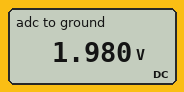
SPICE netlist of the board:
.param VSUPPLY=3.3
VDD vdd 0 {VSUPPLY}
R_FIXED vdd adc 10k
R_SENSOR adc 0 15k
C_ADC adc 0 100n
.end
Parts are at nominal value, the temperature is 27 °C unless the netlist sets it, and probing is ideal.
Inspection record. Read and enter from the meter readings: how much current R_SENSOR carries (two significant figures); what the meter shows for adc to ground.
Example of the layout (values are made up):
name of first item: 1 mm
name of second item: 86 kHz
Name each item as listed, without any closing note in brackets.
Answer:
how much current R_SENSOR carries: 130 µA
what the meter shows for adc to ground: 1.980 V
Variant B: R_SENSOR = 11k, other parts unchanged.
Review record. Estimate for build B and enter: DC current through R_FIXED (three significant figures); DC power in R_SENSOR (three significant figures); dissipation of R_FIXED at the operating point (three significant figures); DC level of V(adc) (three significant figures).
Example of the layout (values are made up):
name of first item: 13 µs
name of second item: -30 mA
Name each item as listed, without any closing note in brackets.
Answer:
DC current through R_FIXED: 157 µA
DC power in R_SENSOR: 272 µW
dissipation of R_FIXED at the operating point: 247 µW
DC level of V(adc): 1.73 V
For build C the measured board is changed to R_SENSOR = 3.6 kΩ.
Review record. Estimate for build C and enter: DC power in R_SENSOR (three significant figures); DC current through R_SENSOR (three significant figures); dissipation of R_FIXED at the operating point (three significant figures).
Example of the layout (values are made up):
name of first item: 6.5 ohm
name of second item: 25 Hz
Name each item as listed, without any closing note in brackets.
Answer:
DC power in R_SENSOR: 212 µW
DC current through R_SENSOR: 243 µA
dissipation of R_FIXED at the operating point: 589 µW
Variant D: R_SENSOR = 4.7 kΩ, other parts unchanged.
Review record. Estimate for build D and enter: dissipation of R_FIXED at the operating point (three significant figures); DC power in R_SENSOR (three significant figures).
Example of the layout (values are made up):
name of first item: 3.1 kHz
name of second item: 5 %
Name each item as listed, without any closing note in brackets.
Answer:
dissipation of R_FIXED at the operating point: 504 µW
DC power in R_SENSOR: 237 µW
